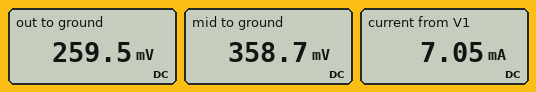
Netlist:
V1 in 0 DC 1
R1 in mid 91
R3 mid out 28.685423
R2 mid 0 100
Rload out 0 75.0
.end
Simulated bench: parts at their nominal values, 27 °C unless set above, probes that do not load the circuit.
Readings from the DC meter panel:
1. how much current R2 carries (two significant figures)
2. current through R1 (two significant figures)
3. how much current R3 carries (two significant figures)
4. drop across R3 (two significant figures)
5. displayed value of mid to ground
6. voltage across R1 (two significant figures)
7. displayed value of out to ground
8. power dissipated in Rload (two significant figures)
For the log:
3.6 mA
7.0 mA
3.5 mA
99 mV
358.7 mV
640 mV
259.5 mV
900 µW
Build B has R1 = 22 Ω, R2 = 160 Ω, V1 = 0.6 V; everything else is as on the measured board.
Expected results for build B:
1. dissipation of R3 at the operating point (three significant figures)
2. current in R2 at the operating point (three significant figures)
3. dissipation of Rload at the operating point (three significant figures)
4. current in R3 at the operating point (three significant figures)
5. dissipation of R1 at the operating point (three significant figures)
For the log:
527 µW
2.78 mA
1.38 mW
4.29 mA
1.10 mW
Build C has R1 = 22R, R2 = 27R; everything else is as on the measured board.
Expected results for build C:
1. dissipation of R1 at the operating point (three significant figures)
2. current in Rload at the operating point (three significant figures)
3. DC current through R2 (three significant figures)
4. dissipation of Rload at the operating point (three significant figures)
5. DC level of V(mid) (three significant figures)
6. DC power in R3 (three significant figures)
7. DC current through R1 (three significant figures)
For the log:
11.7 mW
4.76 mA
18.3 mA
1.70 mW
493 mV
649 µW
23.0 mA
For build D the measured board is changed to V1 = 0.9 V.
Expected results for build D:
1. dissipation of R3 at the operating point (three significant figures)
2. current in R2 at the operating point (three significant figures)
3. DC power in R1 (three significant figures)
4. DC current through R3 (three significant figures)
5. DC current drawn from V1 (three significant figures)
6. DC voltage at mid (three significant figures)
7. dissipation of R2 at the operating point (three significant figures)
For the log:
278 µW
3.23 mA
3.66 mW
3.11 mA
6.34 mA
323 mV
1.04 mW
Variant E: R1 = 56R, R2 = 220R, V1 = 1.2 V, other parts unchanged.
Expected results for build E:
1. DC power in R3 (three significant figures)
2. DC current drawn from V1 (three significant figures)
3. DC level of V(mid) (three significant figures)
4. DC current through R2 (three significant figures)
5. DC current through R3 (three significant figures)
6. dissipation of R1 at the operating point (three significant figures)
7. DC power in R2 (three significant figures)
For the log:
1.19 mW
9.49 mA
669 mV
3.04 mA
6.45 mA
5.04 mW
2.03 mW
